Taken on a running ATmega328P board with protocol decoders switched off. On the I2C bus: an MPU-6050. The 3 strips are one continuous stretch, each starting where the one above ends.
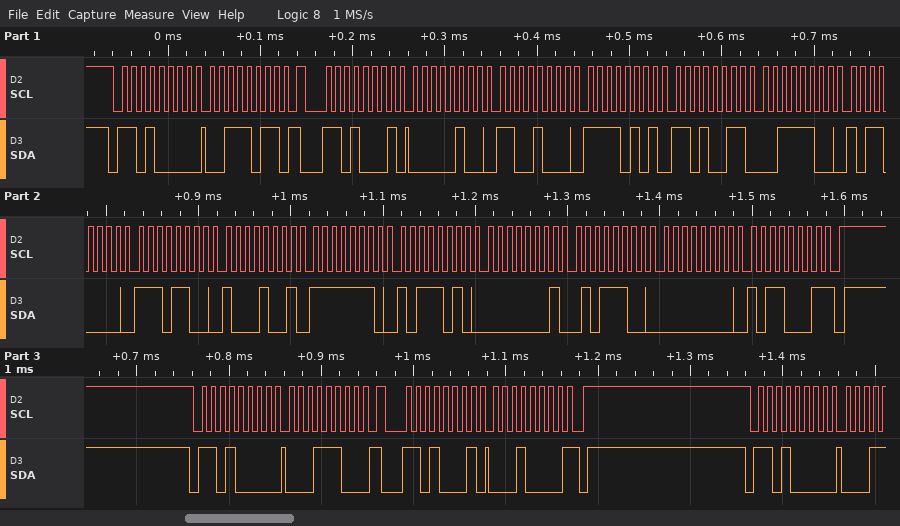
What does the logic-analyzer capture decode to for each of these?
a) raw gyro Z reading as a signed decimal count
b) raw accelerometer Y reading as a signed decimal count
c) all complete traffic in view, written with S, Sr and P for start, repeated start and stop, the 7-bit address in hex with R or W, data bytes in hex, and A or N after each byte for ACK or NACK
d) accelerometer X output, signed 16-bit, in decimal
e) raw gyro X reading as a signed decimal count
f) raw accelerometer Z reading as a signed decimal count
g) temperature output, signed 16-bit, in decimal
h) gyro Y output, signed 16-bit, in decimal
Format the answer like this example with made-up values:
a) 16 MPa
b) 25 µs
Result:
a) 177
b) -2605
c) S 68W A 3B A Sr 68R A 04 A C8 A F5 A D3 A 3C A B0 A EC A 89 A FE A BA A 01 A 5C A 00 A B1 N P S 68W A 1C A Sr 68R A 10 N P S 68W A
d) 1224
e) -326
f) 15536
g) -4983
h) 348
